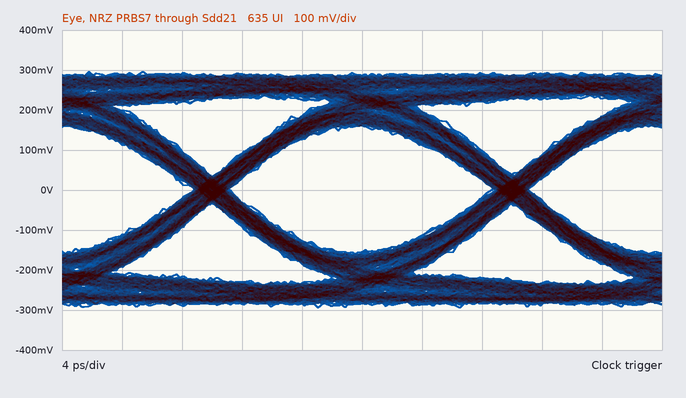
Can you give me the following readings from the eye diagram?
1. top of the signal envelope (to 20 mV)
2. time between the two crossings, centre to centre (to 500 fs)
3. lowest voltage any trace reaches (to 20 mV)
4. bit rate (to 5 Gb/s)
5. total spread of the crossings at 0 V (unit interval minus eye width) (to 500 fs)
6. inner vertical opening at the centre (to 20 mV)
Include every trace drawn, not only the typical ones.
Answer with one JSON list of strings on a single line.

["300 mV", "20.0 ps", "-300 mV", "50 Gb/s", "2.5 ps", "320 mV"]
